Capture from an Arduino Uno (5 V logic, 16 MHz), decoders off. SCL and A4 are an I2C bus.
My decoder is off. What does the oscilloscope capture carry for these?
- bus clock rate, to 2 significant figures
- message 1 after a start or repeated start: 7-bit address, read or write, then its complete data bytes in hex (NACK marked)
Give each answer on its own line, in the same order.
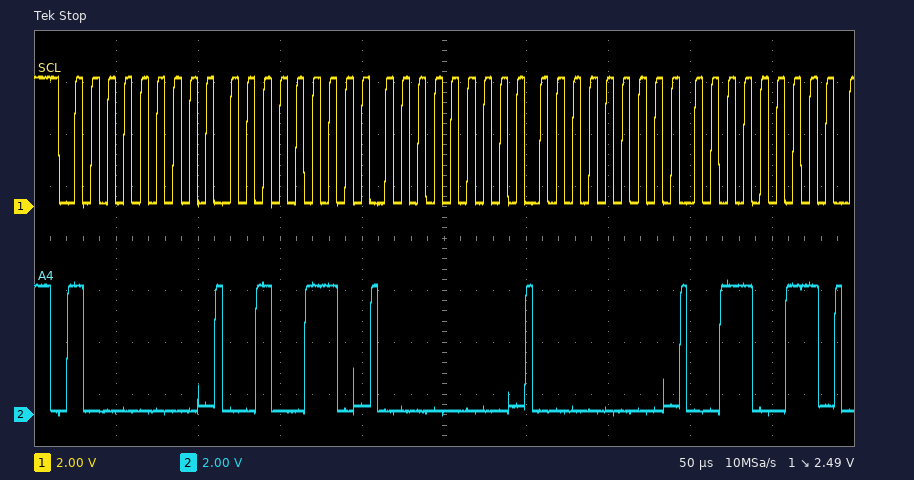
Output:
100 kHz
0x40 write: 26 00 00 33
